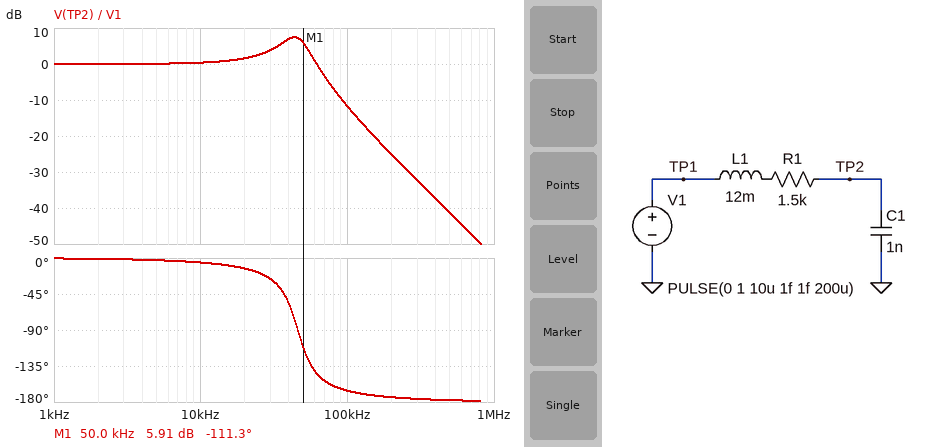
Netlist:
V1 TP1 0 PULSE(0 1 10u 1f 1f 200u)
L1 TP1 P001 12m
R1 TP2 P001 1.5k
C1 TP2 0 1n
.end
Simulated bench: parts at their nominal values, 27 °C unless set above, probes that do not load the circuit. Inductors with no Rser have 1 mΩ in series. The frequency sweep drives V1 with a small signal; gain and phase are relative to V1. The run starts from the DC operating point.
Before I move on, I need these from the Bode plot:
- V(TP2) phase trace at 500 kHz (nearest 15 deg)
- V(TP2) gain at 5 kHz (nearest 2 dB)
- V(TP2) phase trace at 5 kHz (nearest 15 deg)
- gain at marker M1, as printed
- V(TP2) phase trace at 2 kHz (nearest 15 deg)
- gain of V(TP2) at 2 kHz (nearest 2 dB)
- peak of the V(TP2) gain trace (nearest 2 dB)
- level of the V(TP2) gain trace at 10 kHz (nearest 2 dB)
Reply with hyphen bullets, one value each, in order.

- -180 deg
- 0 dB
- 0 deg
- 5.91 dB
- 0 deg
- 0 dB
- 8 dB
- 0 dB
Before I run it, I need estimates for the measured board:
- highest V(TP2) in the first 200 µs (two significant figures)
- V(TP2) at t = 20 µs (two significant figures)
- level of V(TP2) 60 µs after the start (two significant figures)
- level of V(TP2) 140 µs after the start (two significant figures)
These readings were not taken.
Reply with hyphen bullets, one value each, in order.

- 1.5 V
- 1.5 V
- 990 mV
- 1.0 V
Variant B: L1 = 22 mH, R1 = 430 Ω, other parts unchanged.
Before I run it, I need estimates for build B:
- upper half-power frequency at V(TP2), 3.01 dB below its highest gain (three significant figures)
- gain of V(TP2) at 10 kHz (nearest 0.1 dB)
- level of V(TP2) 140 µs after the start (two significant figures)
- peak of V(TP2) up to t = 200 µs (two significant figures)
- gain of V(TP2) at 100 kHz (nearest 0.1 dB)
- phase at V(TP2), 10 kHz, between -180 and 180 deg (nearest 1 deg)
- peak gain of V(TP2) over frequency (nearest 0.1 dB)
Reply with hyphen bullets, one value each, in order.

- 35.4 kHz
- 0.8 dB
- 1.2 V
- 1.9 V
- -17.7 dB
- -2 deg
- 20.8 dB
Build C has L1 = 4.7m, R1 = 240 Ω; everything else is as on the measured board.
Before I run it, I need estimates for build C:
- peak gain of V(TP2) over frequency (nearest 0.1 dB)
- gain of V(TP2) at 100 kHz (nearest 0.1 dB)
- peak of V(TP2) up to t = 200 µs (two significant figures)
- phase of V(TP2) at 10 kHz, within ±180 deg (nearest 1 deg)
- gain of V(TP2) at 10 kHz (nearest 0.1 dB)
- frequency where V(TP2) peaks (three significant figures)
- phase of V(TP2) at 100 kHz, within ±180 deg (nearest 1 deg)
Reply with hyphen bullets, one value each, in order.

- 19.1 dB
- 1.2 dB
- 1.8 V
- -1 deg
- 0.2 dB
- 73.2 kHz
- -170 deg
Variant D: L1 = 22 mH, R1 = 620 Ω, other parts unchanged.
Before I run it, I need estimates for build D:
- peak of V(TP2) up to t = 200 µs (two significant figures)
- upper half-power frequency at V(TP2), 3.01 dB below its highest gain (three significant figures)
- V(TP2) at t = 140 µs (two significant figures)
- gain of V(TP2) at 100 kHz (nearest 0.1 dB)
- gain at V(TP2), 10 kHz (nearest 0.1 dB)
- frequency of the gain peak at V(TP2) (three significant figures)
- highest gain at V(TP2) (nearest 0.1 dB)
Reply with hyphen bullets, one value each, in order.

- 1.8 V
- 36.0 kHz
- 1.1 V
- -17.7 dB
- 0.8 dB
- 33.8 kHz
- 17.6 dB
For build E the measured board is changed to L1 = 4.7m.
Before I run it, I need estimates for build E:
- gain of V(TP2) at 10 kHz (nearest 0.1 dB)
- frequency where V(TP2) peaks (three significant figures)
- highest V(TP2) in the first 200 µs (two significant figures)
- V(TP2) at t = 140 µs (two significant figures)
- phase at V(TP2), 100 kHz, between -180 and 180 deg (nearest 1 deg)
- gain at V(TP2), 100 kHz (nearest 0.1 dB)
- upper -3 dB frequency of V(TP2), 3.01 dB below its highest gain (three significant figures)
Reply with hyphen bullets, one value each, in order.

- 0.1 dB
- 64.0 kHz
- 1.3 V
- 1.0 V
- -132 deg
- -2.1 dB
- 87.2 kHz
